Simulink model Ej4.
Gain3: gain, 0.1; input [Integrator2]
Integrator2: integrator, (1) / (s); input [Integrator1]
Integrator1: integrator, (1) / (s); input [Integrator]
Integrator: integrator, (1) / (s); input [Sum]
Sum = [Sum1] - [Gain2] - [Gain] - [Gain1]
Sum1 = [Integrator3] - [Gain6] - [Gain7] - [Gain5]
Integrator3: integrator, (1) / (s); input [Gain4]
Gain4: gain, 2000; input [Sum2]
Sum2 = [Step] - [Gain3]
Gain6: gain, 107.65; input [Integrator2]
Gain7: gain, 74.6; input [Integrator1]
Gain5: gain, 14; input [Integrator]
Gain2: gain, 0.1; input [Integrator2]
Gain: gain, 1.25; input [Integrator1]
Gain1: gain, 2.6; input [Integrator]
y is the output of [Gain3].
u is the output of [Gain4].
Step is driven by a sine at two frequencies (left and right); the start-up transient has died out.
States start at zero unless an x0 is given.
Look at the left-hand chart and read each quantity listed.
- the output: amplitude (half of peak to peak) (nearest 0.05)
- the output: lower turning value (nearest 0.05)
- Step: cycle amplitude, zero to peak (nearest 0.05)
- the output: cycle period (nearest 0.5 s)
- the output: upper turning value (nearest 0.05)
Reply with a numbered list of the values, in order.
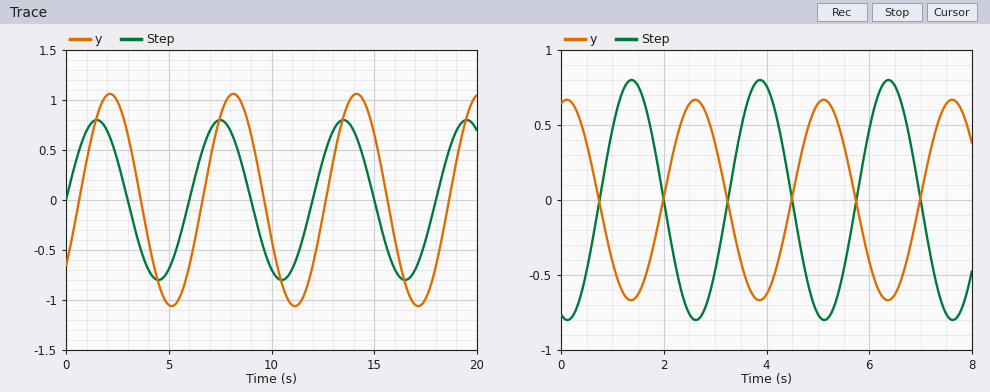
1. 1.05
2. -1.05
3. 0.80
4. 6.0 s
5. 1.05
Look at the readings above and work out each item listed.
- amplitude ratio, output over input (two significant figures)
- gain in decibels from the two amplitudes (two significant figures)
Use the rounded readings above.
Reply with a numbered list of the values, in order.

1. 1.3
2. 2.4 dB
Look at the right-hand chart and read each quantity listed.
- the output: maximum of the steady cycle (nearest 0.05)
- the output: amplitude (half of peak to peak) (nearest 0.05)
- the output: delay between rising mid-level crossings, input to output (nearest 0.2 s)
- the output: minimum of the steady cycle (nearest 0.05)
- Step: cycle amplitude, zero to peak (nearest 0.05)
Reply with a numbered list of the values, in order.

1. 0.65
2. 0.65
3. 1.2 s
4. -0.65
5. 0.80
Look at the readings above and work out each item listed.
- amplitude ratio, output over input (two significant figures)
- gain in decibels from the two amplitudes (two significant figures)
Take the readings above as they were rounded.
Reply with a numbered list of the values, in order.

1. 0.81
2. -1.8 dB
